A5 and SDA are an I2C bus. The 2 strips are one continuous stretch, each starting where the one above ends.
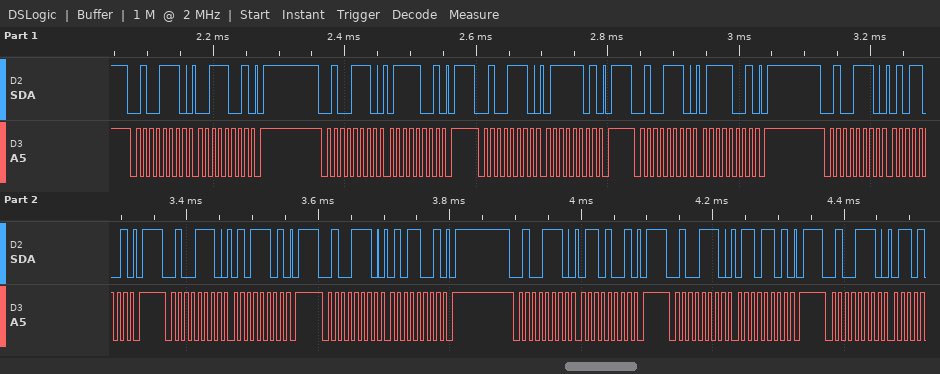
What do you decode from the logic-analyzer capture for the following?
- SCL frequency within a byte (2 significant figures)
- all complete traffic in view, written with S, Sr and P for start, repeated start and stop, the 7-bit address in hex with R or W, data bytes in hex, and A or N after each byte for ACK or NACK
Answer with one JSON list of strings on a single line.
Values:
["100 kHz", "S 27W A 39 A P S 27W A 79 A P S 27W A 7D A P S 27W A 79 A P S 27W A 59 A P S 27W A 5D A P S 27W A 59 A P S 27W A 69 A P S 27W A 6D A P S 27W A"]
